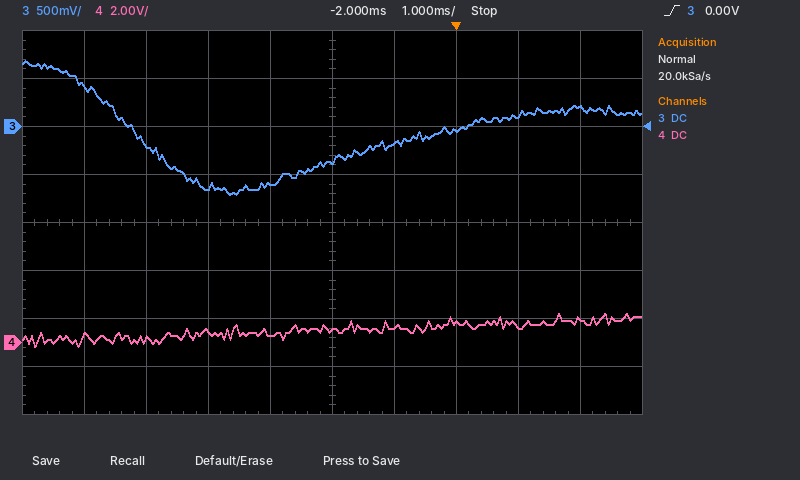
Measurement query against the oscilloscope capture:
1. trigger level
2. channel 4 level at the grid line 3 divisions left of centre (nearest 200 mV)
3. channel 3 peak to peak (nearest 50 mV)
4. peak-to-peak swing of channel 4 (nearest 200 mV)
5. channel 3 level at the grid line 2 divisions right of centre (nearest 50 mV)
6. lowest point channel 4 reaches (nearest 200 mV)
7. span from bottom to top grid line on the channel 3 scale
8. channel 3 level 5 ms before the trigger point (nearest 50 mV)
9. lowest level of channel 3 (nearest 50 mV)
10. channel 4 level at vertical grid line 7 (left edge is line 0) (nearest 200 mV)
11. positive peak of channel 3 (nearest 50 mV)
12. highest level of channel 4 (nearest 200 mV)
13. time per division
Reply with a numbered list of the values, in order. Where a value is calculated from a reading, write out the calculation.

1. 0.00 V
2. 200 mV
3. 700 mV − (-700 mV) = 1.40 V
4. 1.2 V − (-200 mV) = 1.4 V
5. -50 mV
6. -200 mV
7. 4 V
8. -200 mV
9. -700 mV
10. 800 mV
11. 700 mV
12. 1.2 V
13. 1 ms
